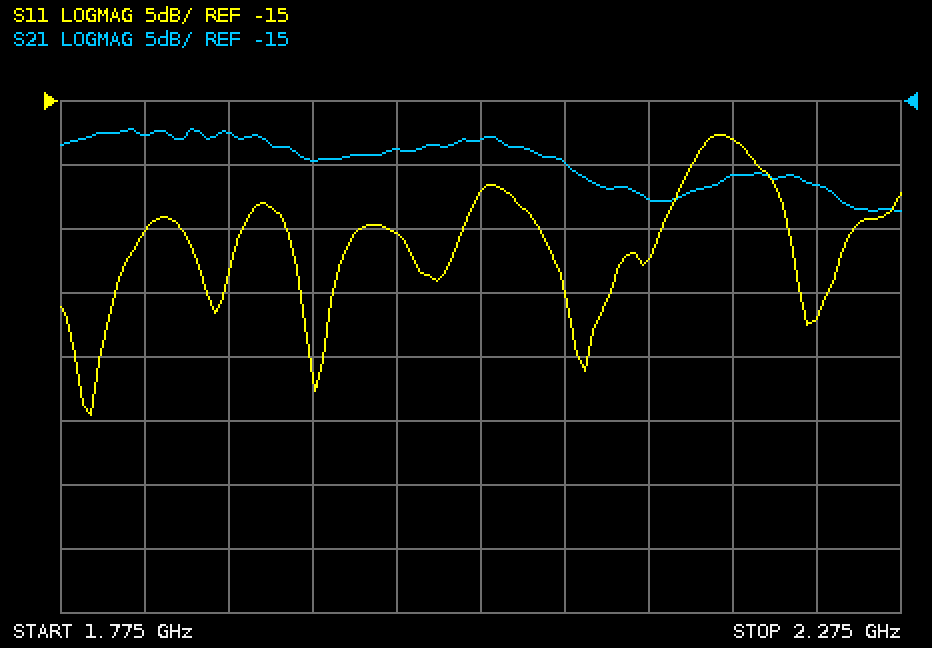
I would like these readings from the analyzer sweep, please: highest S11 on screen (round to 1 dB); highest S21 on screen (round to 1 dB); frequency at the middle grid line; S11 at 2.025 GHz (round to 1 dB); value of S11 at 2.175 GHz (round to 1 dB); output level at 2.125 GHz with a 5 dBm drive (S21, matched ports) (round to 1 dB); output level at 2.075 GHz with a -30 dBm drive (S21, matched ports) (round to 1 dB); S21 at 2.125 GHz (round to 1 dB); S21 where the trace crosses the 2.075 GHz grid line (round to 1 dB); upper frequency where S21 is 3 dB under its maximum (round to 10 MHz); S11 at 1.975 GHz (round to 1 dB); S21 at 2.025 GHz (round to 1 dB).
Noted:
-18 dB
-17 dB
2.025 GHz
-22 dB
-18 dB
-18 dBm
-50 dBm
-23 dB
-20 dB
2.08 GHz
-25 dB
-18 dB
